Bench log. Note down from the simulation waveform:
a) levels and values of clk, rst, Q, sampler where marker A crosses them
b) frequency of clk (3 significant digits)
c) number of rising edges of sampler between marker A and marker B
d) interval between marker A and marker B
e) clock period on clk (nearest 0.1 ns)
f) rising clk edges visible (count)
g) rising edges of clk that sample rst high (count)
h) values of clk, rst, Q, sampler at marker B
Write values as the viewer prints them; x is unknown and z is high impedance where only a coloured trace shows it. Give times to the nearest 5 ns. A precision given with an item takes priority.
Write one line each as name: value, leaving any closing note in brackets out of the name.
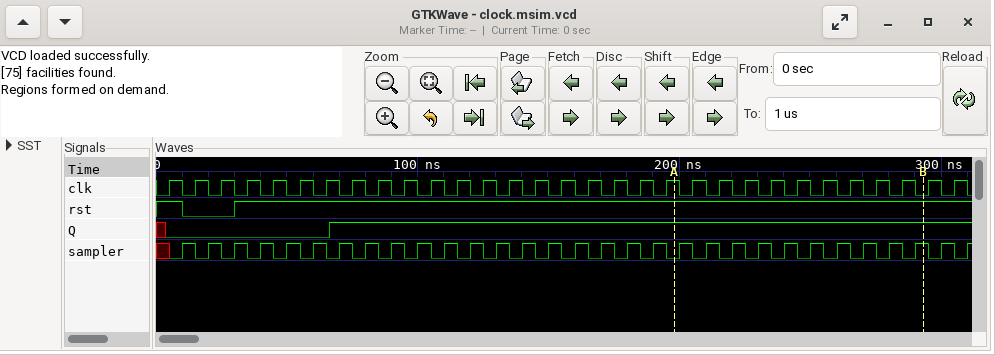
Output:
levels and values of clk, rst, Q, sampler where marker A crosses them: clk=1, rst=1, Q=1, sampler=0
frequency of clk: 100 MHz
number of rising edges of sampler between marker A and marker B: 10
interval between marker A and marker B: 95 ns
clock period on clk: 10 ns
rising clk edges visible: 31
rising edges of clk that sample rst high: 29
values of clk, rst, Q, sampler at marker B: clk=0, rst=1, Q=1, sampler=1
